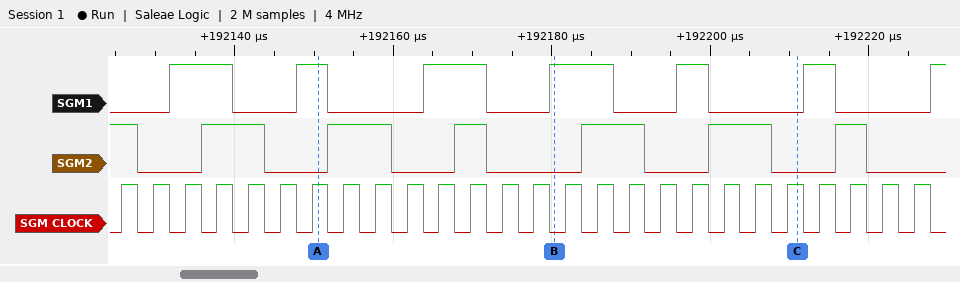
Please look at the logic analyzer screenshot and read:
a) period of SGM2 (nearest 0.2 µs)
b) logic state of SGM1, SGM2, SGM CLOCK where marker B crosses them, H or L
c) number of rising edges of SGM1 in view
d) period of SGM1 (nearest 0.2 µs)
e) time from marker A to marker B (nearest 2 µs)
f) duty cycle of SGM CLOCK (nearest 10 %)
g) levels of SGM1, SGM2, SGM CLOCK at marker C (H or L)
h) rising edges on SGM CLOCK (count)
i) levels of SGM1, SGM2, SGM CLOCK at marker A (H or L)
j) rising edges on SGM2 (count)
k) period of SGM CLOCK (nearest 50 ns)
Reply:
16 µs
SGM1=H, SGM2=L, SGM CLOCK=L
7
16 µs
30 µs
50 %
SGM1=L, SGM2=L, SGM CLOCK=H
26
SGM1=H, SGM2=L, SGM CLOCK=H
6
4000 ns
